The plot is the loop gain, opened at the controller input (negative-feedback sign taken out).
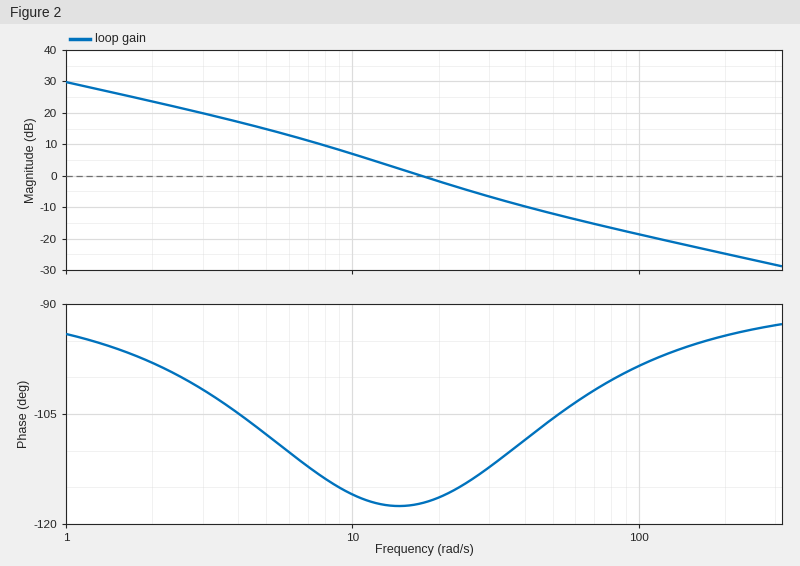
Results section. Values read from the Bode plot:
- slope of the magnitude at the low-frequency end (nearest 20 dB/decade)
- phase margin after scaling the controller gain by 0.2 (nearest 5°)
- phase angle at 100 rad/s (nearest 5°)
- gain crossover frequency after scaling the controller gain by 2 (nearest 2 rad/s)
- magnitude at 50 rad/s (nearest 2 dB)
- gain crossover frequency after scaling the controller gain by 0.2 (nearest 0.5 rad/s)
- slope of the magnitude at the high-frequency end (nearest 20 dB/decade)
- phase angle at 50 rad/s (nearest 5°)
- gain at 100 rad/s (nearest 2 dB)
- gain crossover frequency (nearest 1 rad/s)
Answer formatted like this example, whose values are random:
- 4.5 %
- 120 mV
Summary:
- -20 dB/decade
- 70°
- -100°
- 28 rad/s
- -12 dB
- 5.5 rad/s
- -20 dB/decade
- -105°
- -18 dB
- 17 rad/s
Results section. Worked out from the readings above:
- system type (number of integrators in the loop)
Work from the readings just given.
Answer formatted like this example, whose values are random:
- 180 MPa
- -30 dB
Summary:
- 1
